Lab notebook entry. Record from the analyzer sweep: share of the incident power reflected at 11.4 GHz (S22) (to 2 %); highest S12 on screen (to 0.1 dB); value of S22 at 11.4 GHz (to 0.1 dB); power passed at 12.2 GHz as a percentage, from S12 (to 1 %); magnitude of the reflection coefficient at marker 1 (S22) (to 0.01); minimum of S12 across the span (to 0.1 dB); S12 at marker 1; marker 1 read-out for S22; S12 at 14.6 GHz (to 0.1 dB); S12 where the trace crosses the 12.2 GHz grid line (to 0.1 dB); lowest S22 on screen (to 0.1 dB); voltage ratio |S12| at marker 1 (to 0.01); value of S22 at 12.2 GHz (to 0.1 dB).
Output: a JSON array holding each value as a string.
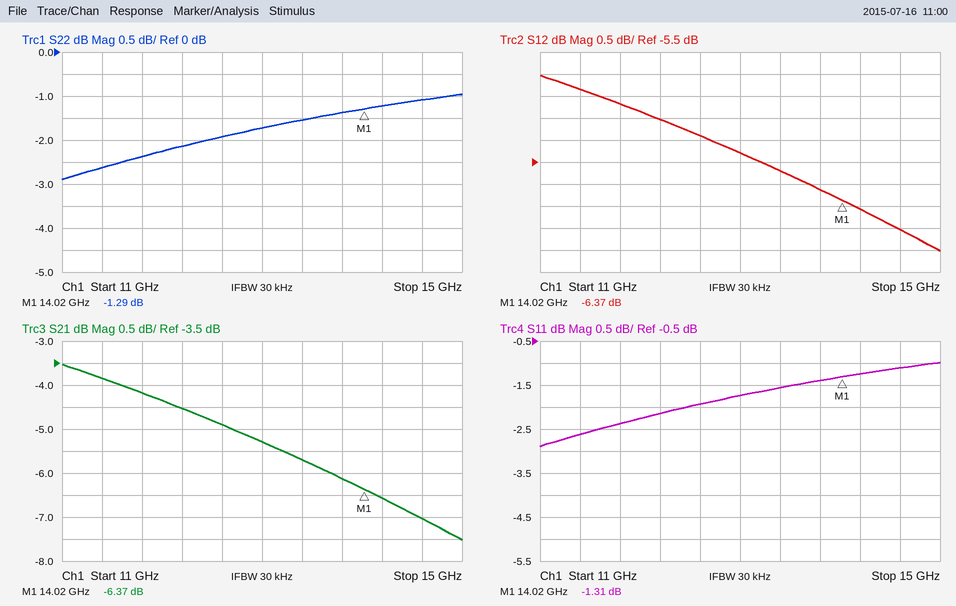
["54 %", "-3.5 dB", "-2.6 dB", "35 %", "0.86", "-7.5 dB", "-6.37 dB", "-1.29 dB", "-7.0 dB", "-4.5 dB", "-2.9 dB", "0.48", "-2.1 dB"]
